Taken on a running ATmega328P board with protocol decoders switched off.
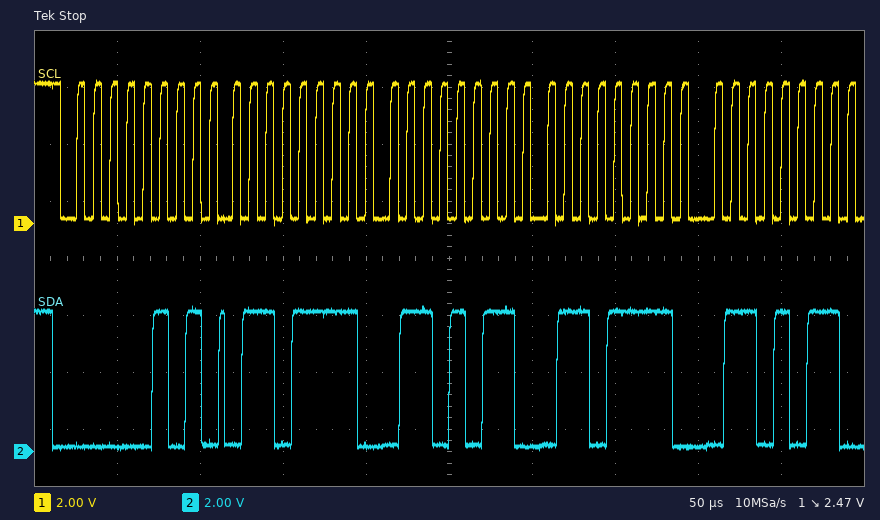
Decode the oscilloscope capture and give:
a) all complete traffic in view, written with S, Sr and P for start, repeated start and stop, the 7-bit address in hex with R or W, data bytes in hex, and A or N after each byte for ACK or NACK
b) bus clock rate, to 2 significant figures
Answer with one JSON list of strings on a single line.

["S 02R A 6F A 6B A 6F A 6B A", "100 kHz"]
